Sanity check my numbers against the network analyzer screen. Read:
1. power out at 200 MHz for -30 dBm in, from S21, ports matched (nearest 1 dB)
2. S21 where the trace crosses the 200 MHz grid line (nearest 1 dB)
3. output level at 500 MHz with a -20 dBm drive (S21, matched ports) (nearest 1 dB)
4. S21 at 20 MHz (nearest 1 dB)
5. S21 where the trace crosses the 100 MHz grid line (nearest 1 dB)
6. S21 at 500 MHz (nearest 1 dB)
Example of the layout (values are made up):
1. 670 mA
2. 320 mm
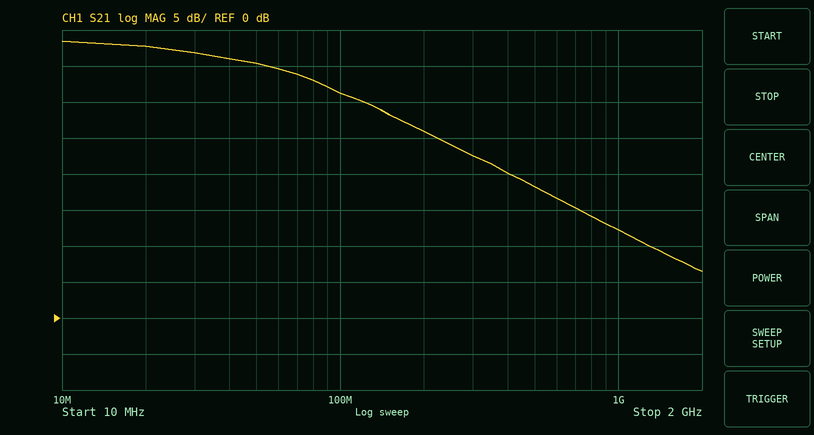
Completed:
1. -4 dBm
2. 26 dB
3. -2 dBm
4. 38 dB
5. 31 dB
6. 18 dB
